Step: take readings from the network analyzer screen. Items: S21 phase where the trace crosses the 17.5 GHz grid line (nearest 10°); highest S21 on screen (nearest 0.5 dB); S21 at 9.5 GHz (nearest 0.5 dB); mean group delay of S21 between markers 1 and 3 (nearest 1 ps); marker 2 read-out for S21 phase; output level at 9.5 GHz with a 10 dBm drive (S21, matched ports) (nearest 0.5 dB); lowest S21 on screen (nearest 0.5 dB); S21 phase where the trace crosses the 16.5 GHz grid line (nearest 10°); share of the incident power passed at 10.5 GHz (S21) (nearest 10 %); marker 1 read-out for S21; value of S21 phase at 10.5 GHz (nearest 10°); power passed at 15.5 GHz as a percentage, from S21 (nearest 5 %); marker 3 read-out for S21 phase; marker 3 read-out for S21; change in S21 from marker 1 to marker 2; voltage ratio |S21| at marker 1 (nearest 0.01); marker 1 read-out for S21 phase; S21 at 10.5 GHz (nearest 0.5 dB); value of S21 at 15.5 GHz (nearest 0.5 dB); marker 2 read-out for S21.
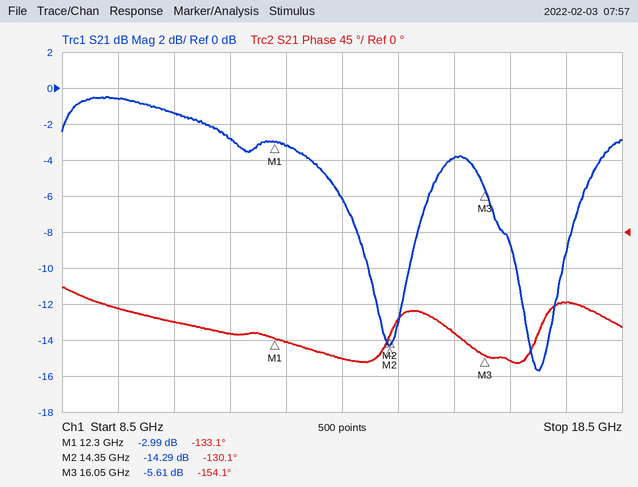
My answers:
-90°
-0.5 dB
-0.5 dB
16 ps
-130.1°
9.5 dBm
-15.5 dB
-160°
70 %
-2.99 dB
-110°
40 %
-154.1°
-5.61 dB
-11.30 dB
0.71
-133.1°
-1.5 dB
-4.0 dB
-14.29 dB
